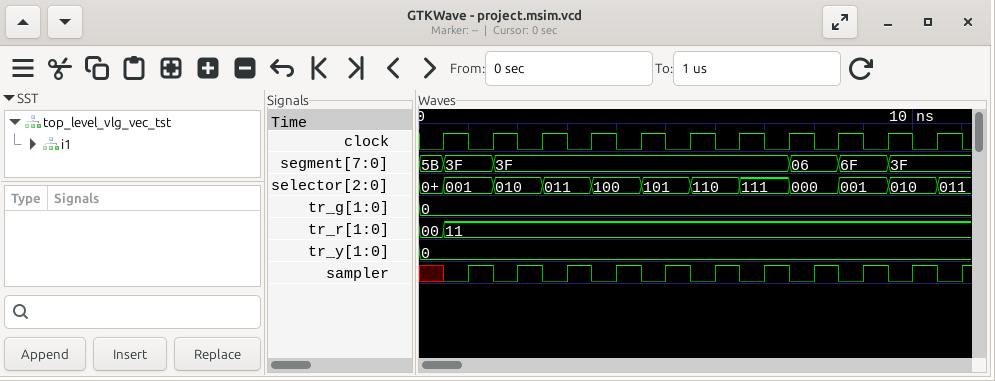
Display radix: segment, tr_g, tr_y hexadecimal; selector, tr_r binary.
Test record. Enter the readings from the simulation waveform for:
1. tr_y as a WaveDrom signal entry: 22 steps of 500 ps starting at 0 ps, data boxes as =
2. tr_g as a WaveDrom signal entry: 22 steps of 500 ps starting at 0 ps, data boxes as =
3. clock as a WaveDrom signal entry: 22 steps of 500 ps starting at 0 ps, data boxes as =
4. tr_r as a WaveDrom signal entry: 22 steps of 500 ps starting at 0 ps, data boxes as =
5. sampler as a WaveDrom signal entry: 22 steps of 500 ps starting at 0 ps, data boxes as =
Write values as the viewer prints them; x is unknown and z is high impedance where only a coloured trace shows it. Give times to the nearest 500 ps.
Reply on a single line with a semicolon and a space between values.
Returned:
{name: 'tr_y', wave: '=.....................', data: '0'}; {name: 'tr_g', wave: '=.....................', data: '0'}; {name: 'clock', wave: '0101010101010101010101'}; {name: 'tr_r', wave: '==....................', data: '00 11'}; {name: 'sampler', wave: 'x010101010101010101010'}
